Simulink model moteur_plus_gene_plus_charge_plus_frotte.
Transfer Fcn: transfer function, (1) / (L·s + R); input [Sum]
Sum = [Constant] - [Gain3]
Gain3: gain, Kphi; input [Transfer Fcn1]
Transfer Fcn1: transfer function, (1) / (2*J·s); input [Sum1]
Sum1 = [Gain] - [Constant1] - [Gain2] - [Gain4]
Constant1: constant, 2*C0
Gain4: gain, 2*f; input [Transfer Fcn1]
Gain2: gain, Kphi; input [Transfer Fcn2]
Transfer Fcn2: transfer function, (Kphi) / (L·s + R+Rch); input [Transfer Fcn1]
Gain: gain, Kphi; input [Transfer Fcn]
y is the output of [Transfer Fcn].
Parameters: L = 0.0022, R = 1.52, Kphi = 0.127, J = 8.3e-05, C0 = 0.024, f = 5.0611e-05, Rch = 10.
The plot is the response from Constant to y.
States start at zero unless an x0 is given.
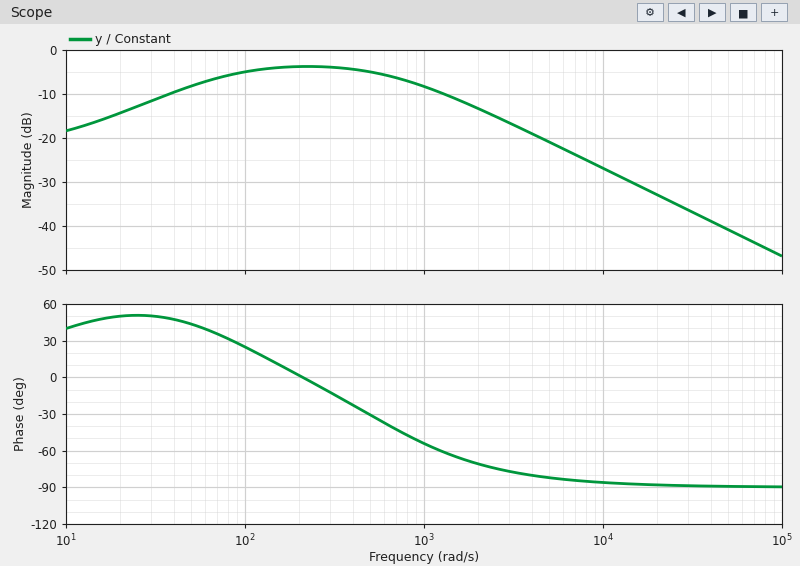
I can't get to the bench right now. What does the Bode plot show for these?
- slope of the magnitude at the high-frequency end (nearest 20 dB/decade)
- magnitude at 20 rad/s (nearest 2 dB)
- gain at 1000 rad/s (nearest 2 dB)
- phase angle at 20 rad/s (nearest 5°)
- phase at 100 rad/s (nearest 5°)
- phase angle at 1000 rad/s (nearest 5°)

-20 dB/decade
-14 dB
-8 dB
50°
25°
-55°
